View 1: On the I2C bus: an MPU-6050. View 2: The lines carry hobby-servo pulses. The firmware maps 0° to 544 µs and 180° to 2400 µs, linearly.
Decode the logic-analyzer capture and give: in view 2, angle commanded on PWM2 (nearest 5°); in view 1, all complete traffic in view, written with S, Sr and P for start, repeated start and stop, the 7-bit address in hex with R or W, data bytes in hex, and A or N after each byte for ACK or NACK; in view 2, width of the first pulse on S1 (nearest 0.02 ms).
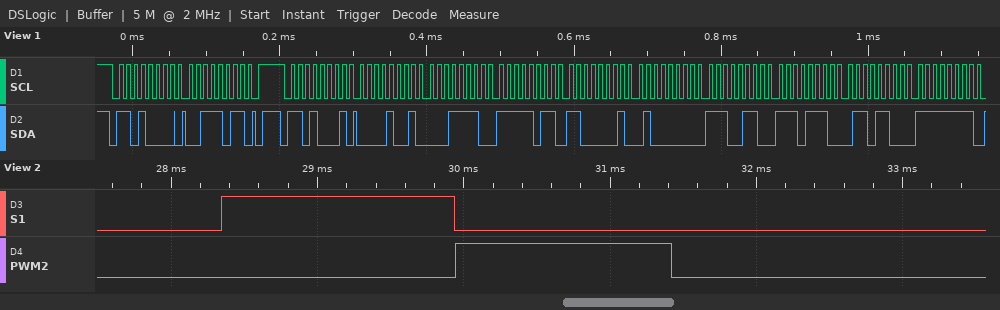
90°
S 68W A 3B A P S 68R A 09 A 1E A FB A C1 A 40 A E6 A EE A 6C A FF A
1.60 ms
